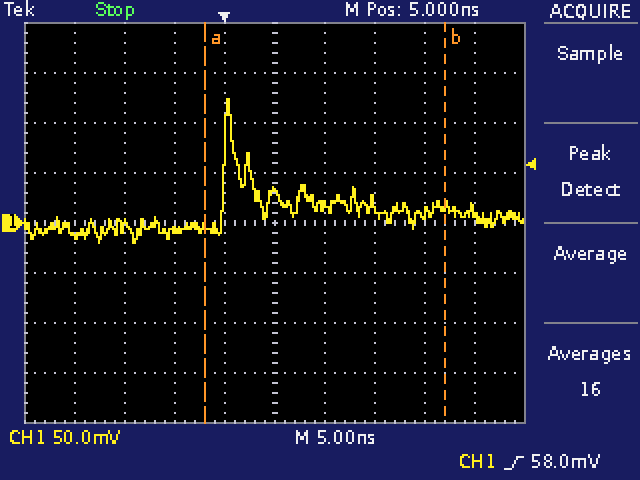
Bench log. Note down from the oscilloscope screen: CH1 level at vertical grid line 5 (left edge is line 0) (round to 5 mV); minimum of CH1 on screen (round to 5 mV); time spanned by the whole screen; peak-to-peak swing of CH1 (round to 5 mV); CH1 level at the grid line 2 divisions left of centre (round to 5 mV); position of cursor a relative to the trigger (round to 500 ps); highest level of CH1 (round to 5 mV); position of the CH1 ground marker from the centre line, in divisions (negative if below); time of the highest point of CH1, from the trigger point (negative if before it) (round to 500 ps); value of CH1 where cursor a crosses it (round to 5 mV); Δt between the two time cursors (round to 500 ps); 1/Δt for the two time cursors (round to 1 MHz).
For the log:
30 mV
-20 mV
50 ns
145 mV
-5 mV
-2.0 ns
125 mV
0.0 div
+500 ps
-5 mV
24.0 ns
42 MHz
